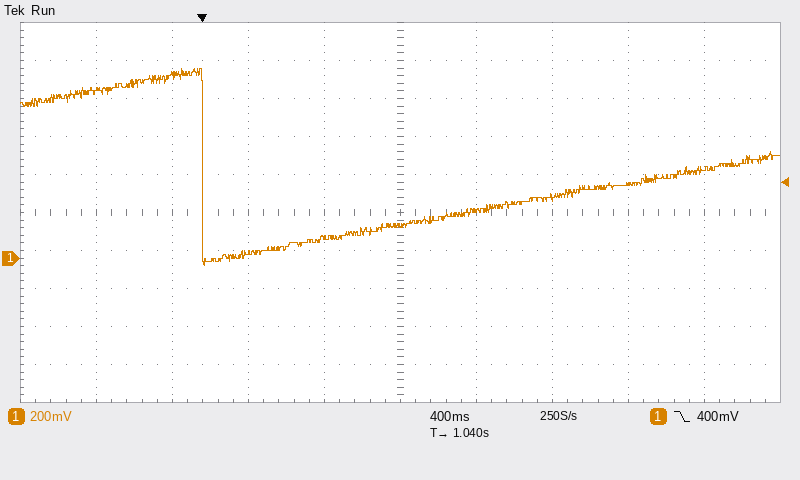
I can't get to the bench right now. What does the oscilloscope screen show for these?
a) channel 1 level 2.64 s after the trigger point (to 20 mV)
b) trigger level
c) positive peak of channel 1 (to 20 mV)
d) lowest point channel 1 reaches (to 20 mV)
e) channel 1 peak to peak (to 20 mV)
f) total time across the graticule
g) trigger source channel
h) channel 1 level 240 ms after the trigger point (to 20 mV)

460 mV
400 mV
1.00 V
-40 mV
1.04 V
4 s
channel 1
20 mV
